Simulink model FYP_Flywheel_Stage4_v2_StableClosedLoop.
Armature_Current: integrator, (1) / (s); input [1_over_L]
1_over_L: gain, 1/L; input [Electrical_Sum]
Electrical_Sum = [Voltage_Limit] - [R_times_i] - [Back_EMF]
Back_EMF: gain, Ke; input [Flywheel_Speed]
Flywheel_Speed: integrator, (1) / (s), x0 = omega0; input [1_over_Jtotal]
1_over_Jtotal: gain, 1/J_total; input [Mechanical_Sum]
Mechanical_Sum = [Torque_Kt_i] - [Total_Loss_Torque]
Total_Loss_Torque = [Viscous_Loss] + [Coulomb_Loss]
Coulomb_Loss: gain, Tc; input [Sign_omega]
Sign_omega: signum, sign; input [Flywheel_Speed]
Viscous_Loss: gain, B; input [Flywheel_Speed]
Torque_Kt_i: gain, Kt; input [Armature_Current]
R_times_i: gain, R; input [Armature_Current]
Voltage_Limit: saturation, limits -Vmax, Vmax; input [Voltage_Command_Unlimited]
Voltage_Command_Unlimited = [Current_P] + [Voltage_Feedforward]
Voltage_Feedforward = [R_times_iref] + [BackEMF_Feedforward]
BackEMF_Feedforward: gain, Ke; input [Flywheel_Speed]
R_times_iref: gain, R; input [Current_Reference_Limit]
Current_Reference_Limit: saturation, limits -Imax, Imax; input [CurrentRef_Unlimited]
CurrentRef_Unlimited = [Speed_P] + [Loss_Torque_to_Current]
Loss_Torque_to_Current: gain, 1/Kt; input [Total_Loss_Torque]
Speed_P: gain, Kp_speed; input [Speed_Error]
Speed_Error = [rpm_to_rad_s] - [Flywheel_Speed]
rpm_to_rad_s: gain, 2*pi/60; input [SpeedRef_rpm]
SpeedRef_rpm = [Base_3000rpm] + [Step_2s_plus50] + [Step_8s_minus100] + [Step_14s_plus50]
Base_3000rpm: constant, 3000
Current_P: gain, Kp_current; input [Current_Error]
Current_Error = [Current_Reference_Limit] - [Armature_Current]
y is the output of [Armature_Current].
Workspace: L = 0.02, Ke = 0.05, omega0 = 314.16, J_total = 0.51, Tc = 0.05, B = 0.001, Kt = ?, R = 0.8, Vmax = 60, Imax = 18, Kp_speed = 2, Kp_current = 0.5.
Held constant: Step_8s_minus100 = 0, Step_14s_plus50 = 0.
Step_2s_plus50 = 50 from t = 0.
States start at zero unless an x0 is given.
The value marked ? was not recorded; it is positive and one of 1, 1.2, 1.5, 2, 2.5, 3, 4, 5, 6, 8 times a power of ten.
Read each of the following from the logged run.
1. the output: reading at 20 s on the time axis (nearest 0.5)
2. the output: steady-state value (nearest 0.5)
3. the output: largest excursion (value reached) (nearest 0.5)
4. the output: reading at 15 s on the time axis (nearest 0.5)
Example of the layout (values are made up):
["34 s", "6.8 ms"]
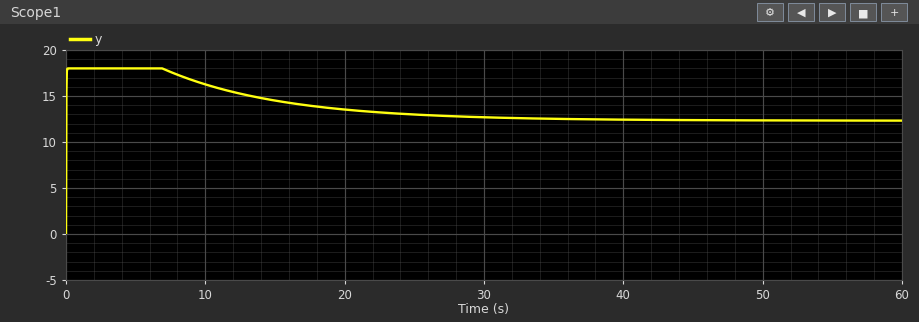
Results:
["13.5", "12.5", "18.0", "14.5"]
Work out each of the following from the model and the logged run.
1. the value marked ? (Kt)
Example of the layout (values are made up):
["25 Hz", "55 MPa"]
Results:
["0.03"]
